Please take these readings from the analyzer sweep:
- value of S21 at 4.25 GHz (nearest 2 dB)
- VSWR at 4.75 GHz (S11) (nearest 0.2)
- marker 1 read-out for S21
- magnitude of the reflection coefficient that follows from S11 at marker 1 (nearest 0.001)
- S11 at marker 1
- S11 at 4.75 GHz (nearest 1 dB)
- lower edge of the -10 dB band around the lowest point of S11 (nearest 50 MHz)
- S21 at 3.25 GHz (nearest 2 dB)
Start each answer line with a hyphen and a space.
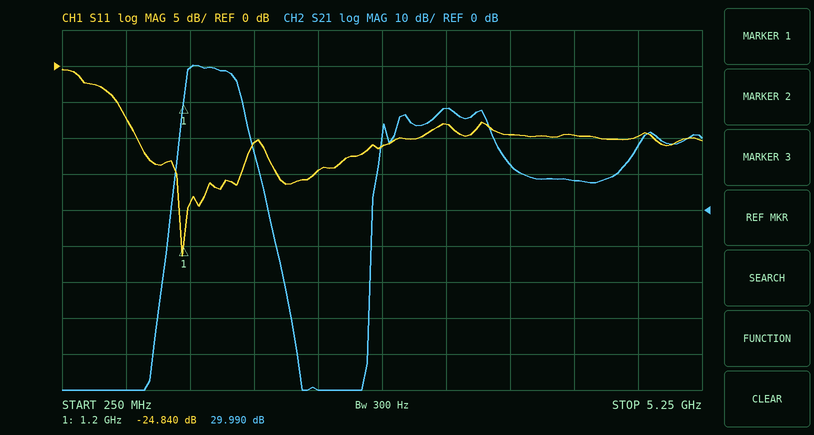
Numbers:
- 8 dB
- 2.0
- 29.990 dB
- 0.057
- -24.840 dB
- -10 dB
- 850 MHz
- 28 dB
